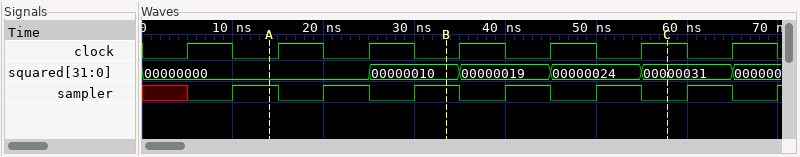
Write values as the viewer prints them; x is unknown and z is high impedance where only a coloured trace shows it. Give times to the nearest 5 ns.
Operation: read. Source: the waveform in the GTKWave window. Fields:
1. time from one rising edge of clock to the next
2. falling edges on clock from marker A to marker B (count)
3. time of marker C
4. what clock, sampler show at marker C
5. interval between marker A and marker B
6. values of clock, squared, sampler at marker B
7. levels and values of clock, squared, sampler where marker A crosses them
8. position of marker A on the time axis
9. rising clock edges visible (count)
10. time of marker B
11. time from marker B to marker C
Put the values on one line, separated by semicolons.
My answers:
10 ns; 2; 60 ns; clock=1, sampler=0; 20 ns; clock=0, squared=00000010, sampler=1; clock=0, squared=00000000, sampler=1; 15 ns; 7; 35 ns; 25 ns
